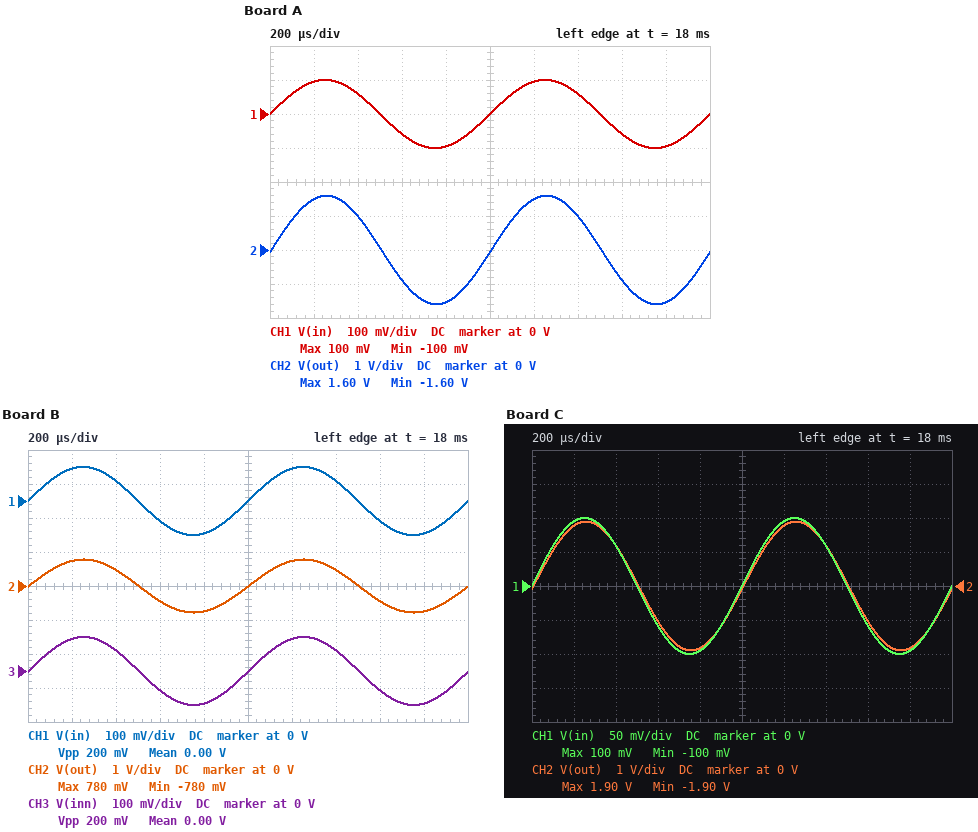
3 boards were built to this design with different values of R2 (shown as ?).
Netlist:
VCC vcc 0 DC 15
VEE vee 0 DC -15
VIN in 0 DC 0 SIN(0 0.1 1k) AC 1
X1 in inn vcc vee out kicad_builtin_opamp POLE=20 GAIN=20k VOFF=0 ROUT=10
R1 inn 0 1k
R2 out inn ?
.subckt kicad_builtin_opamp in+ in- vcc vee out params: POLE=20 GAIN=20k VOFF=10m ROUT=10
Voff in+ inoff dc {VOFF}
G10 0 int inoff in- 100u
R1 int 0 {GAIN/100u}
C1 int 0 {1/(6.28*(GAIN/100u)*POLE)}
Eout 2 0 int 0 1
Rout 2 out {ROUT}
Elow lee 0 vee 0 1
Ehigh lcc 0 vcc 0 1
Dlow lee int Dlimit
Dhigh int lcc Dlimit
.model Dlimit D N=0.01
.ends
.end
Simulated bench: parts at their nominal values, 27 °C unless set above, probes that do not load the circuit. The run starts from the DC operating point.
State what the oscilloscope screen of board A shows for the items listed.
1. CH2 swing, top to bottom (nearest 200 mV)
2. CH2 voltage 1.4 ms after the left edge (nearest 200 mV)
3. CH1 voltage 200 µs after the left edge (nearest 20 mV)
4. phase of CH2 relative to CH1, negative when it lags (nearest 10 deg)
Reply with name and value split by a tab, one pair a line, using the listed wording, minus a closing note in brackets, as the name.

CH2 swing, top to bottom	3.2 V
CH2 voltage 1.4 ms after the left edge	1.0 V
CH1 voltage 200 µs after the left edge	100 mV
phase of CH2 relative to CH1, negative when it lags	0 deg
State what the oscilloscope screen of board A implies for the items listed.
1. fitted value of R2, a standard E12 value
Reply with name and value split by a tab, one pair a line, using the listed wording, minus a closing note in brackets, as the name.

fitted value of R2, a standard E12 value	15 kΩ
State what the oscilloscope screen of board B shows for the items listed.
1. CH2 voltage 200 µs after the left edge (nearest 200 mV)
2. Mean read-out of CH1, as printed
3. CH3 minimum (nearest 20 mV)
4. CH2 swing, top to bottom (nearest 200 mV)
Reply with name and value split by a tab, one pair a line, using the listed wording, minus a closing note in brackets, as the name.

CH2 voltage 200 µs after the left edge	800 mV
Mean read-out of CH1, as printed	0.00 V
CH3 minimum	-100 mV
CH2 swing, top to bottom	1.6 V
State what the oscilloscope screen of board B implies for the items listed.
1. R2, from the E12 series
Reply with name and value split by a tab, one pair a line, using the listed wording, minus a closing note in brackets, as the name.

R2, from the E12 series	6.8 kΩ
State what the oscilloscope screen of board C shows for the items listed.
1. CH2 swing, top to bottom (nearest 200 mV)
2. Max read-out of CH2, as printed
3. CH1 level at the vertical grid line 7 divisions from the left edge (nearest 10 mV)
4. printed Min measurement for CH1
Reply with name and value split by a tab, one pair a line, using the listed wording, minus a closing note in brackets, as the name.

CH2 swing, top to bottom	3.8 V
Max read-out of CH2, as printed	1.90 V
CH1 level at the vertical grid line 7 divisions from the left edge	60 mV
printed Min measurement for CH1	-100 mV
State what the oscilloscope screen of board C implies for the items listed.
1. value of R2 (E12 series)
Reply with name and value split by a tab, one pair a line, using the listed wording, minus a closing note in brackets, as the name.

value of R2	18 kΩ
